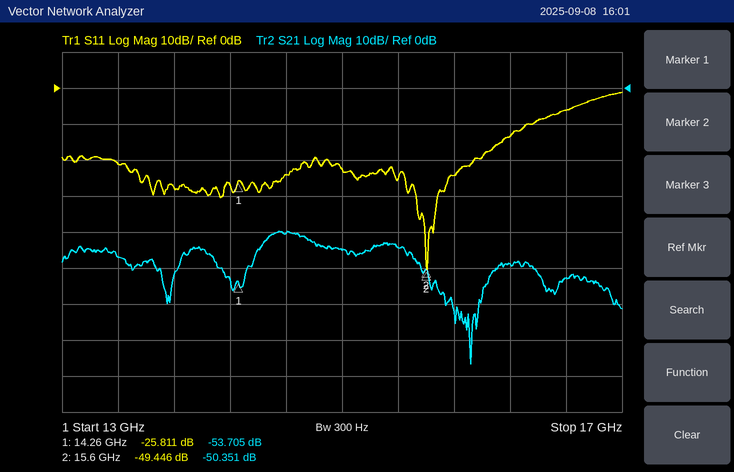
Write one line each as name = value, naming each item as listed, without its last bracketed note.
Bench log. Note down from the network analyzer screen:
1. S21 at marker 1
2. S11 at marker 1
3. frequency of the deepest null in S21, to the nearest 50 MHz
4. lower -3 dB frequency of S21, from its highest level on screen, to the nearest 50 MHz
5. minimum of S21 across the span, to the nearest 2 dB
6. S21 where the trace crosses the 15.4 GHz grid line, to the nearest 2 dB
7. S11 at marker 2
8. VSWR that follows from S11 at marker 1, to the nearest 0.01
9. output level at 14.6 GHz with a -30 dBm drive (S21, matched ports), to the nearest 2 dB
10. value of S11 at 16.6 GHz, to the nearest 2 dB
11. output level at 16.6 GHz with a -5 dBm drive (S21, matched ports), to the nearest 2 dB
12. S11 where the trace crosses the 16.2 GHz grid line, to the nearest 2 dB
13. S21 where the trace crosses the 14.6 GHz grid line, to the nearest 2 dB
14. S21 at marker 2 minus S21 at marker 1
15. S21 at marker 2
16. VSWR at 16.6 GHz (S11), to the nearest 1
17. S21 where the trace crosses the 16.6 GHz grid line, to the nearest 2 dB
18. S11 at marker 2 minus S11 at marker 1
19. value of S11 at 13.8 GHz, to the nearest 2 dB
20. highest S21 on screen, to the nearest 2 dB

S21 at marker 1 = -53.705 dB
S11 at marker 1 = -25.811 dB
frequency of the deepest null in S21, to the nearest 50 MHz = 15.90 GHz
lower -3 dB frequency of S21, from its highest level on screen, to the nearest 50 MHz = 14.45 GHz
minimum of S21 across the span, to the nearest 2 dB = -76 dB
S21 where the trace crosses the 15.4 GHz grid line, to the nearest 2 dB = -44 dB
S11 at marker 2 = -49.446 dB
VSWR that follows from S11 at marker 1, to the nearest 0.01 = 1.11
output level at 14.6 GHz with a -30 dBm drive (S21, matched ports), to the nearest 2 dB = -70 dBm
value of S11 at 16.6 GHz, to the nearest 2 dB = -6 dB
output level at 16.6 GHz with a -5 dBm drive (S21, matched ports), to the nearest 2 dB = -58 dBm
S11 where the trace crosses the 16.2 GHz grid line, to the nearest 2 dB = -14 dB
S21 where the trace crosses the 14.6 GHz grid line, to the nearest 2 dB = -40 dB
S21 at marker 2 minus S21 at marker 1 = 3.354 dB
S21 at marker 2 = -50.351 dB
VSWR at 16.6 GHz (S11), to the nearest 1 = 3
S21 where the trace crosses the 16.6 GHz grid line, to the nearest 2 dB = -52 dB
S11 at marker 2 minus S11 at marker 1 = -23.635 dB
value of S11 at 13.8 GHz, to the nearest 2 dB = -28 dB
highest S21 on screen, to the nearest 2 dB = -40 dB
